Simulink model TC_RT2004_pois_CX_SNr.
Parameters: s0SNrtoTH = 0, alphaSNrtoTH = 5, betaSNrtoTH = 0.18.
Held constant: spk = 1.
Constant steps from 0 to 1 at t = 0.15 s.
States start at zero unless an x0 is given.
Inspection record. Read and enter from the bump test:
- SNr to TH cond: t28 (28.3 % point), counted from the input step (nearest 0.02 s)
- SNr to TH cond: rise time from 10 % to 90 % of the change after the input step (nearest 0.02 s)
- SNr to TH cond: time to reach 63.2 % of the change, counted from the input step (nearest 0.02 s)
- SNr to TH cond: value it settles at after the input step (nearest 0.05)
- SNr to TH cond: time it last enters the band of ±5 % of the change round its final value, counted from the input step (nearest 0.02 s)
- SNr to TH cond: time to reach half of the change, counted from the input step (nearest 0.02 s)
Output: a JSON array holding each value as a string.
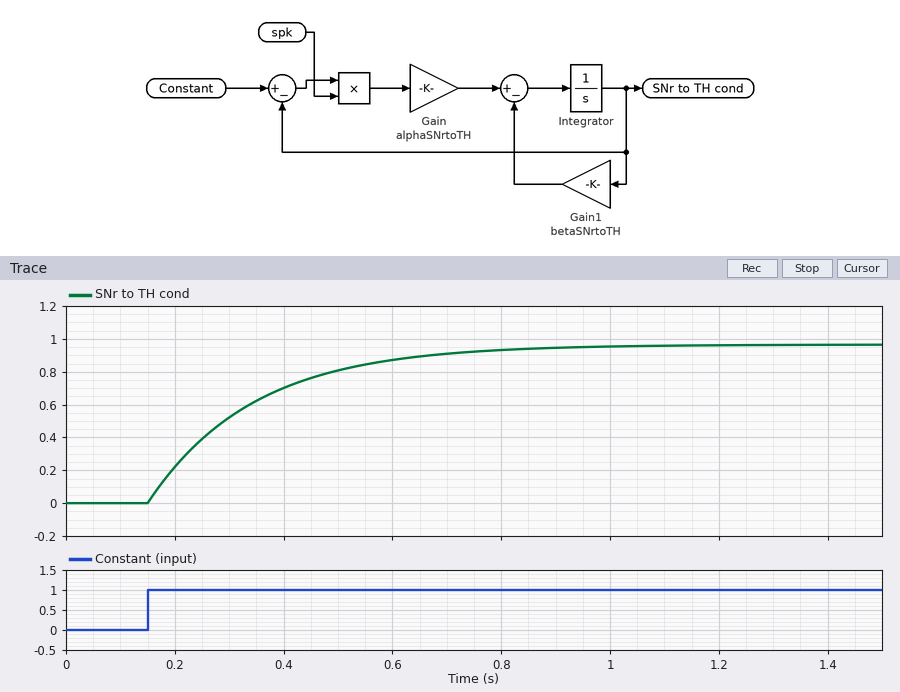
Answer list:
["0.06 s", "0.42 s", "0.20 s", "0.95", "0.58 s", "0.14 s"]
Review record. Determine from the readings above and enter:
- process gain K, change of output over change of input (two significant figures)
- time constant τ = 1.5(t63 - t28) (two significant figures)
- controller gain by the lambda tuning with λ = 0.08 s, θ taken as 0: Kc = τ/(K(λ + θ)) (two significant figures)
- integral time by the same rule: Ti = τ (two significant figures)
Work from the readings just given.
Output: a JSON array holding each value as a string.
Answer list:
["0.95", "0.21 s", "2.8", "0.21 s"]
